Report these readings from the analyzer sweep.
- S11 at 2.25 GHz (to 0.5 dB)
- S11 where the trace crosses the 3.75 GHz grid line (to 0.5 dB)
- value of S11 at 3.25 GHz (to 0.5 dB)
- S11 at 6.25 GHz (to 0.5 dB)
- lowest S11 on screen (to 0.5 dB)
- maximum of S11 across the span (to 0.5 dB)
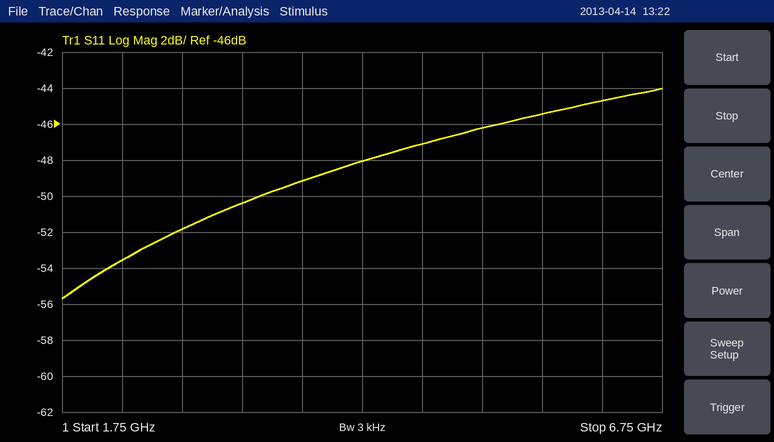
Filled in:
-53.5 dB
-49.0 dB
-50.5 dB
-44.5 dB
-55.5 dB
-44.0 dB
